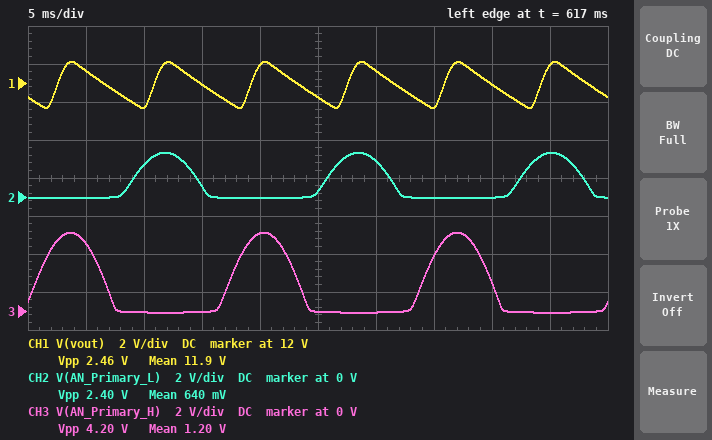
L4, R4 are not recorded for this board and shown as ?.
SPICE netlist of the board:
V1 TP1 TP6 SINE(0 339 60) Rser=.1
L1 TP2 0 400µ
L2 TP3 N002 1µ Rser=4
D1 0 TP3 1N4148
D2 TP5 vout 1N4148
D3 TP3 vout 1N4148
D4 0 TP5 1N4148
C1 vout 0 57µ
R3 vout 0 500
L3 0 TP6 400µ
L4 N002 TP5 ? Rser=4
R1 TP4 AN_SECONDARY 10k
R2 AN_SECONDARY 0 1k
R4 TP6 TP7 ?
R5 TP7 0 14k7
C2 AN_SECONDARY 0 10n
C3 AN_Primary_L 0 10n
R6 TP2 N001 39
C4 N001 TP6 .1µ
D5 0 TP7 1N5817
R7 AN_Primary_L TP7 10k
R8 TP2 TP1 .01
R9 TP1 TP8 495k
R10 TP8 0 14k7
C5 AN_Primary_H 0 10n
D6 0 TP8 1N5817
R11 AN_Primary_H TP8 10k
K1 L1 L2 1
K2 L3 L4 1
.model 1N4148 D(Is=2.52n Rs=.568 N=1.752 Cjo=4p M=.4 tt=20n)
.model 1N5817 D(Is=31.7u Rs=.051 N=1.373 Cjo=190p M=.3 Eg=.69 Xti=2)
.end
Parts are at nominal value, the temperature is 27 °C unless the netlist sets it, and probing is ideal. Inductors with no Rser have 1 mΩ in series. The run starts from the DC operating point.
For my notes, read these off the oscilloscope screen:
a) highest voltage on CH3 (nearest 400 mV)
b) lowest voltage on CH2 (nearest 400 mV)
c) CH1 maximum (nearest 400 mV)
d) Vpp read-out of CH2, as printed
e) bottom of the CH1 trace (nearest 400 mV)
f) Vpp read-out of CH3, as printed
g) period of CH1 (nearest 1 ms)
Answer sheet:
4.0 V
0 V
13.2 V
2.40 V
10.8 V
4.20 V
8 ms
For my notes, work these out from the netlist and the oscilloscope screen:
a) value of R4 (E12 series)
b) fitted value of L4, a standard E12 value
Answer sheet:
820 kΩ
820 nH
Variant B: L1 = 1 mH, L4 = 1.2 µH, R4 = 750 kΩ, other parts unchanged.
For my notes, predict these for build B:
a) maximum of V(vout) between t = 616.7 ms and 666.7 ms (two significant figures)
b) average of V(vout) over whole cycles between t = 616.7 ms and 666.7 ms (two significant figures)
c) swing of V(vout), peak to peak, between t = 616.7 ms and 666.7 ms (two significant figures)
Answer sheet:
11 V
9.8 V
2.0 V
